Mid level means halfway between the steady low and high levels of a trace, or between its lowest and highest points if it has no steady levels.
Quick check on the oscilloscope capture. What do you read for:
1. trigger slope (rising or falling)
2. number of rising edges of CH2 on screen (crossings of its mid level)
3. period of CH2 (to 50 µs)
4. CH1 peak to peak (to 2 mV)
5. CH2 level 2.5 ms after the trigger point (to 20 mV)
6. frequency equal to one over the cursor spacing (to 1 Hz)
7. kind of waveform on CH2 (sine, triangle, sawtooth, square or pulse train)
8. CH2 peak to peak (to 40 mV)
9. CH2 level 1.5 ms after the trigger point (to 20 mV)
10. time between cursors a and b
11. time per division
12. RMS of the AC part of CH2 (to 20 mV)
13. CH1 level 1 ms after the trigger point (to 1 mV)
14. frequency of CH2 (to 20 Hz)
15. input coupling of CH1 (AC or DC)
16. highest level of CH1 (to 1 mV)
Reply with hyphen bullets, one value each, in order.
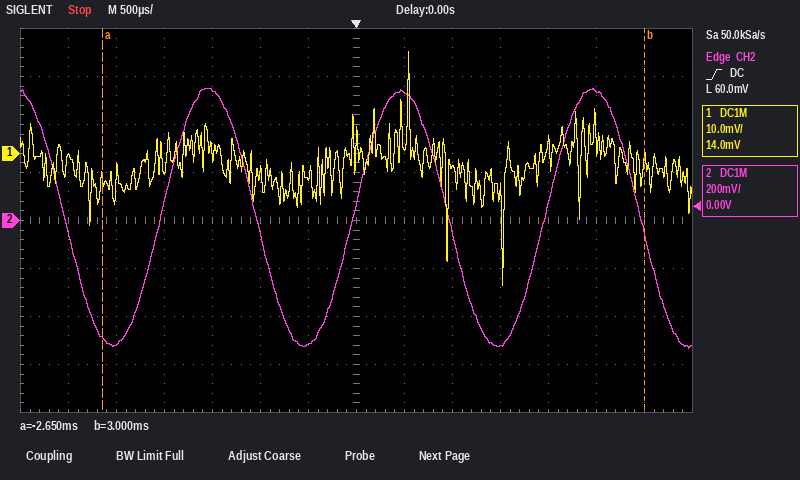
- rising
- 3
- 2.00 ms
- 48 mV
- 540 mV
- 177 Hz
- sine
- 1.08 V
- -520 mV
- 5.65 ms
- 500 µs
- 380 mV
- -3 mV
- 500 Hz
- DC
- 21 mV
